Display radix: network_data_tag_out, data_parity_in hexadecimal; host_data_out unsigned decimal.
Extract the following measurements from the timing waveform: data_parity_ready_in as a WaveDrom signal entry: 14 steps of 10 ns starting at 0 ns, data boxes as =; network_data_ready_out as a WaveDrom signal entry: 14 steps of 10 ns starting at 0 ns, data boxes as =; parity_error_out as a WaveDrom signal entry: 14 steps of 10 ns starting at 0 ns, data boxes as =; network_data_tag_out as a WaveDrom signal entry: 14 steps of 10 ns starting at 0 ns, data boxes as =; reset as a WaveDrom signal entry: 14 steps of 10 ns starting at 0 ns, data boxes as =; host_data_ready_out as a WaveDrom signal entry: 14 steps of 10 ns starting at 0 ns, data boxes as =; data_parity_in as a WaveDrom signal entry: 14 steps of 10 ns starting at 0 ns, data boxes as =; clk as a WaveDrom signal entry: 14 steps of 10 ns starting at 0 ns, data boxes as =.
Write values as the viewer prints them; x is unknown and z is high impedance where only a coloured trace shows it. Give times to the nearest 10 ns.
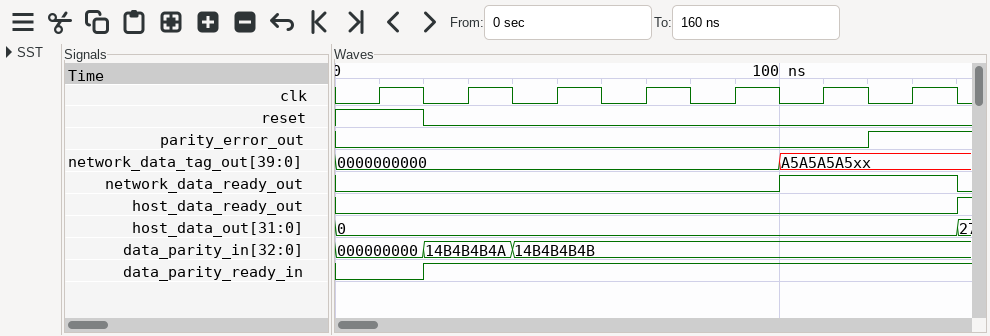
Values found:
{name: 'data_parity_ready_in', wave: '0.1...........'}
{name: 'network_data_ready_out', wave: '0.........1...'}
{name: 'parity_error_out', wave: '0...........1.'}
{name: 'network_data_tag_out', wave: '=.........=...', data: '0000000000 A5A5A5A5xx'}
{name: 'reset', wave: '1.0...........'}
{name: 'host_data_ready_out', wave: '0.............'}
{name: 'data_parity_in', wave: '=.=.=.........', data: '000000000 14B4B4B4A 14B4B4B4B'}
{name: 'clk', wave: '01010101010101'}
